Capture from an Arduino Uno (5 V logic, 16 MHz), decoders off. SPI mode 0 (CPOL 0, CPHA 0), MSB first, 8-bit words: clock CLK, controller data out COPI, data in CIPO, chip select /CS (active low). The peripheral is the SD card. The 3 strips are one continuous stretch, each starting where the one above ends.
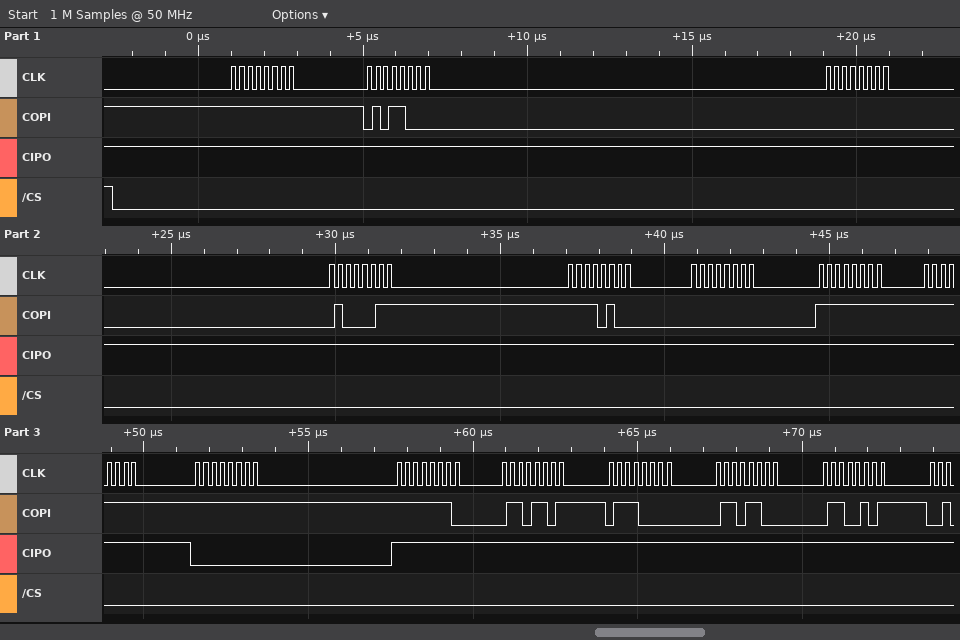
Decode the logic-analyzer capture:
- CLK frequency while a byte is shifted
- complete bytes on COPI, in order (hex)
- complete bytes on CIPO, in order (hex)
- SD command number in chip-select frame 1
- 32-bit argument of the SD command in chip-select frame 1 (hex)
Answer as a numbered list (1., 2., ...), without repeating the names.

1. 4 MHz
2. FF 58 00 43 F4 00 FF FF FF FE 6D 70 6C 65
3. FF FF FF FF FF FF FF FF 00 FF FF FF FF FF
4. CMD24
5. 0x0043F400
